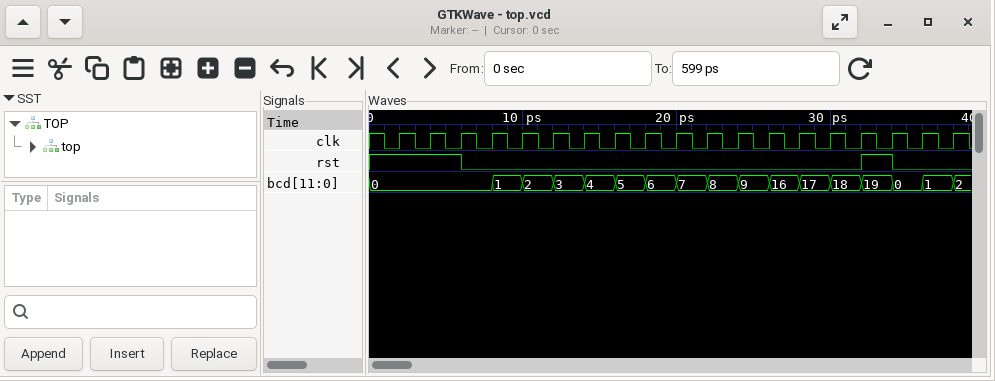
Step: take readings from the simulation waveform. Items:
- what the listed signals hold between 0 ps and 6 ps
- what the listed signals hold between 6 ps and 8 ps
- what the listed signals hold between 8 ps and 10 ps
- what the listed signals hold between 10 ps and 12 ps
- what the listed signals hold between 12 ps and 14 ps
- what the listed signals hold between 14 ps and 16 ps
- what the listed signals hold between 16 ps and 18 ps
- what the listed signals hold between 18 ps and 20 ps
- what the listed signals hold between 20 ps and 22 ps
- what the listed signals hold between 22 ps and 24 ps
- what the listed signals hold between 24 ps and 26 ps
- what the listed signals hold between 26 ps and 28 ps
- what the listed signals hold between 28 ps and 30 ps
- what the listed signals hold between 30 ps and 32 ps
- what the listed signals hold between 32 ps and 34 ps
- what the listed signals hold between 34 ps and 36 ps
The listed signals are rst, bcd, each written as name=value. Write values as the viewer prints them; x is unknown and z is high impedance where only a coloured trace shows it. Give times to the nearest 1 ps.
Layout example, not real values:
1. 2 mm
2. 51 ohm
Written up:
1. rst=1, bcd=0
2. rst=0, bcd=0
3. rst=0, bcd=1
4. rst=0, bcd=2
5. rst=0, bcd=3
6. rst=0, bcd=4
7. rst=0, bcd=5
8. rst=0, bcd=6
9. rst=0, bcd=7
10. rst=0, bcd=8
11. rst=0, bcd=9
12. rst=0, bcd=16
13. rst=0, bcd=17
14. rst=0, bcd=18
15. rst=1, bcd=19
16. rst=0, bcd=0
